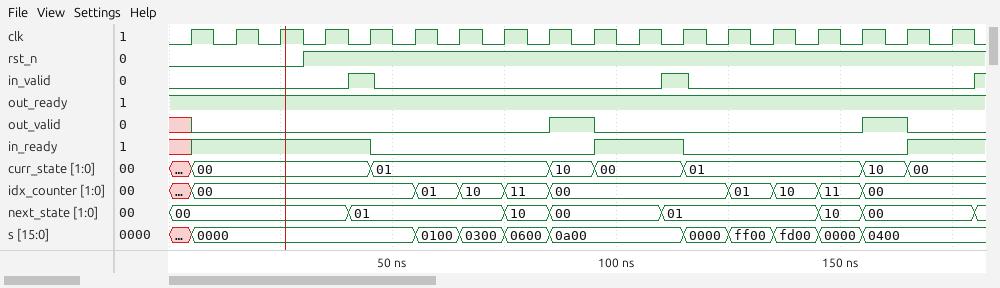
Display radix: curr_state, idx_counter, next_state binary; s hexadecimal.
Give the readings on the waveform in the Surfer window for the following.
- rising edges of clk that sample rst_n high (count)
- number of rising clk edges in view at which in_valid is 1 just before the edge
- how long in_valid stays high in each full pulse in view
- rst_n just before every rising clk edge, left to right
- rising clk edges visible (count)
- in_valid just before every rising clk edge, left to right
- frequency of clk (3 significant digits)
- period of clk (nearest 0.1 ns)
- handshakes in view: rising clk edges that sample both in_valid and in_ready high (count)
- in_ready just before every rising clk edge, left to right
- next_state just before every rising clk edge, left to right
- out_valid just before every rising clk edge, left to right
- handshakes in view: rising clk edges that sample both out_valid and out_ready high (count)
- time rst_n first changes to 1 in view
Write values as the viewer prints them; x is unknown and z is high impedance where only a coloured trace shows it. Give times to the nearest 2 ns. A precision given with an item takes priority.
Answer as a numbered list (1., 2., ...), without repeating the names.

1. 15
2. 2
3. 6 ns, 6 ns
4. 0 0 0 1 1 1 1 1 1 1 1 1 1 1 1 1 1 1
5. 18
6. 0 0 0 0 1 0 0 0 0 0 0 1 0 0 0 0 0 0
7. 100 MHz
8. 10 ns
9. 2
10. x 1 1 1 1 0 0 0 0 0 1 1 0 0 0 0 0 1
11. 00, 00, 00, 00, 01, 01, 01, 01, 10, 00, 00, 01, 01, 01, 01, 10, 00, 00
12. x 0 0 0 0 0 0 0 0 1 0 0 0 0 0 0 1 0
13. 2
14. 30 ns
